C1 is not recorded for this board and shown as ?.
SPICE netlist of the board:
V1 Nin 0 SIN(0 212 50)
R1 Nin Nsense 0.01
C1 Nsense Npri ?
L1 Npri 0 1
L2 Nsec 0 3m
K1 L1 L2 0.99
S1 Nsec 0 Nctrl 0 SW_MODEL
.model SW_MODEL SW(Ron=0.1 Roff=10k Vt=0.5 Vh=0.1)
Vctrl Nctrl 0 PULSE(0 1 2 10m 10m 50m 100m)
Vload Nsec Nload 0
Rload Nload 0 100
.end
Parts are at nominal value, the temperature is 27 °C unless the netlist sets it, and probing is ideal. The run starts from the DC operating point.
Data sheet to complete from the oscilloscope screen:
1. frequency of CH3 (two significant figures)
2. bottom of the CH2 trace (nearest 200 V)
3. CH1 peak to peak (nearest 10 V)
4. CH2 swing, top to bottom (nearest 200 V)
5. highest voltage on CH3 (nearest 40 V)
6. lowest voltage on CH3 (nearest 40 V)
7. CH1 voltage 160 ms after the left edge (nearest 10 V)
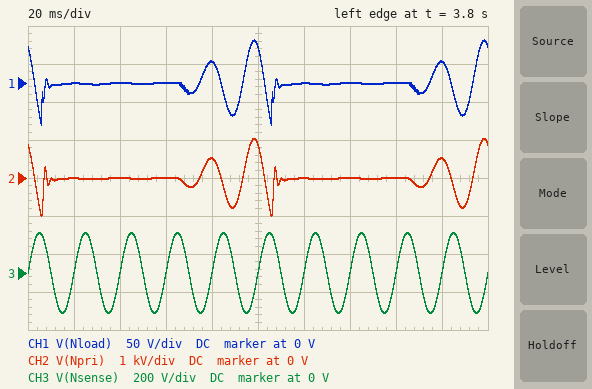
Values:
50 Hz
-1.0 kV
110 V
2.0 kV
200 V
-200 V
0 V
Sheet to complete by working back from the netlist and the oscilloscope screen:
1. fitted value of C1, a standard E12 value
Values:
8.2 µF
